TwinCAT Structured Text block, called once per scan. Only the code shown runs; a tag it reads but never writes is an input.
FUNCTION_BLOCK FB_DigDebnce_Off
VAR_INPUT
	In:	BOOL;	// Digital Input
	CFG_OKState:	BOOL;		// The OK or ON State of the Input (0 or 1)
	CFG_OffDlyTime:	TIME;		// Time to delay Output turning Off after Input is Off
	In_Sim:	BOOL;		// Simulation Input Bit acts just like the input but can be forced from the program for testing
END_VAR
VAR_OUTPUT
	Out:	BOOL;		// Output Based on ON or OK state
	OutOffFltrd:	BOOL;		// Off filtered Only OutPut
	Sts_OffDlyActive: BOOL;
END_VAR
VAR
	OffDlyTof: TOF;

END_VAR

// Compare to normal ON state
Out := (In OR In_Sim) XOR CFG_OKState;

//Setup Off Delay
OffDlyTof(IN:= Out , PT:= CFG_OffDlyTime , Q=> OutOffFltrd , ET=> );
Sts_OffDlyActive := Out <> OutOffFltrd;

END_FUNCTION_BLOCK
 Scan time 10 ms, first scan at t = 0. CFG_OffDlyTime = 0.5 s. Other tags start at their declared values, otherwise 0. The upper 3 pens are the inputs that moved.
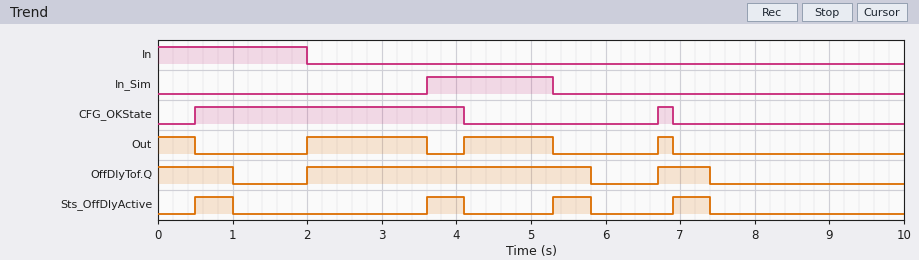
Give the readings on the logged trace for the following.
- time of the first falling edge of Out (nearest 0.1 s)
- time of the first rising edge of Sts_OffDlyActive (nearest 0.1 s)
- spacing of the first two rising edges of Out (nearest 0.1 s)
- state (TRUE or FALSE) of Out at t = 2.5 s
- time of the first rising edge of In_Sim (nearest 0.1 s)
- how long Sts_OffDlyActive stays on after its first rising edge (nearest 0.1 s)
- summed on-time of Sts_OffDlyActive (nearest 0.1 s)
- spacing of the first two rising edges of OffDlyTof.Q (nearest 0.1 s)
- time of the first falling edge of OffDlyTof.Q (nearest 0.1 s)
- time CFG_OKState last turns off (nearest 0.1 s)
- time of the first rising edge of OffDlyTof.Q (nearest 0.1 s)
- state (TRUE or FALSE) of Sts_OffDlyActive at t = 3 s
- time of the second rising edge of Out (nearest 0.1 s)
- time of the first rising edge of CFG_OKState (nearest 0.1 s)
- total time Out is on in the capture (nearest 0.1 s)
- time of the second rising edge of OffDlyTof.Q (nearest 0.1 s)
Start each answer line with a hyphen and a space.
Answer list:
- 0.5 s
- 0.5 s
- 2.1 s
- TRUE
- 3.6 s
- 0.5 s
- 2.0 s
- 4.7 s
- 1.0 s
- 6.9 s
- 2.0 s
- FALSE
- 4.1 s
- 0.5 s
- 3.5 s
- 6.7 s
